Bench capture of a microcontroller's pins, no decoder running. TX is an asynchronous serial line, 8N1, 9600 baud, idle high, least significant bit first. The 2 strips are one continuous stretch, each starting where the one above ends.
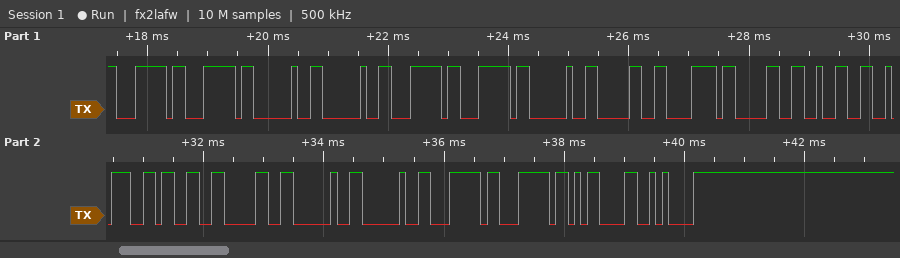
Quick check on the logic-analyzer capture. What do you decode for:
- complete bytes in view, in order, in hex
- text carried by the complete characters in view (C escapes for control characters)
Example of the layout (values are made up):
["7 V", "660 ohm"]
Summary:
["7C 7C 20 20 7C 7C 20 30 78 30 32 3A 33 30 20 20 7C 7C 0D 0A", "\"||  || 0x02:30  ||\\r\\n\""]
